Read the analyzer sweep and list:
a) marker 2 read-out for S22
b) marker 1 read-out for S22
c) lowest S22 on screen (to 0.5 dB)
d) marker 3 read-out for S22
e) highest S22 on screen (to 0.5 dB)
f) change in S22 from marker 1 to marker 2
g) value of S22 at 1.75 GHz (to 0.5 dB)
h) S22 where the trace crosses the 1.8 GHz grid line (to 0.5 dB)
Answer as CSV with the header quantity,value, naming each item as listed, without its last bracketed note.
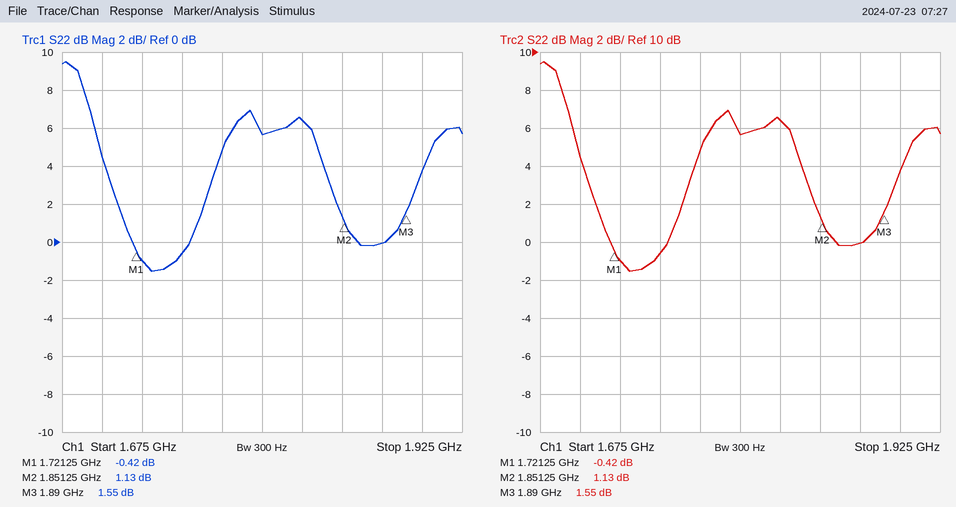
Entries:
quantity,value
marker 2 read-out for S22,1.13 dB
marker 1 read-out for S22,-0.42 dB
lowest S22 on screen,-1.5 dB
marker 3 read-out for S22,1.55 dB
highest S22 on screen,9.5 dB
change in S22 from marker 1 to marker 2,1.55 dB
value of S22 at 1.75 GHz,-0.5 dB
S22 where the trace crosses the 1.8 GHz grid line,5.5 dB
